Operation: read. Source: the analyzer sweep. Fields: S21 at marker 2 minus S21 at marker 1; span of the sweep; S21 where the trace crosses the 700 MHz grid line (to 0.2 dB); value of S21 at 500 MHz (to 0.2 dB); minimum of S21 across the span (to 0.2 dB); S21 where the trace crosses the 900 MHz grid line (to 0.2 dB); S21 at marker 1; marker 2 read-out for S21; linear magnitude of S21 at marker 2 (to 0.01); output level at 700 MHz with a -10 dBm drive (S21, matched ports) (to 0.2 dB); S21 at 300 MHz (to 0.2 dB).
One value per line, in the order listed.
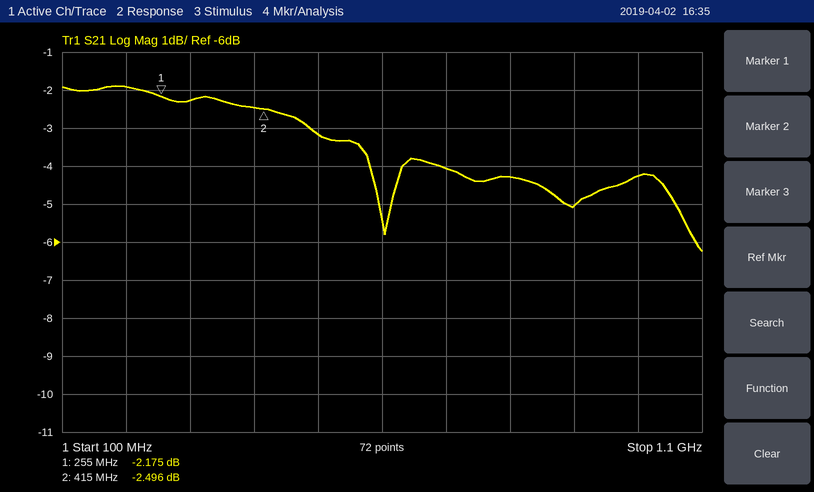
-0.321 dB
1 GHz
-4.0 dB
-3.2 dB
-6.2 dB
-5.0 dB
-2.175 dB
-2.496 dB
0.75
-14.0 dBm
-2.2 dB
